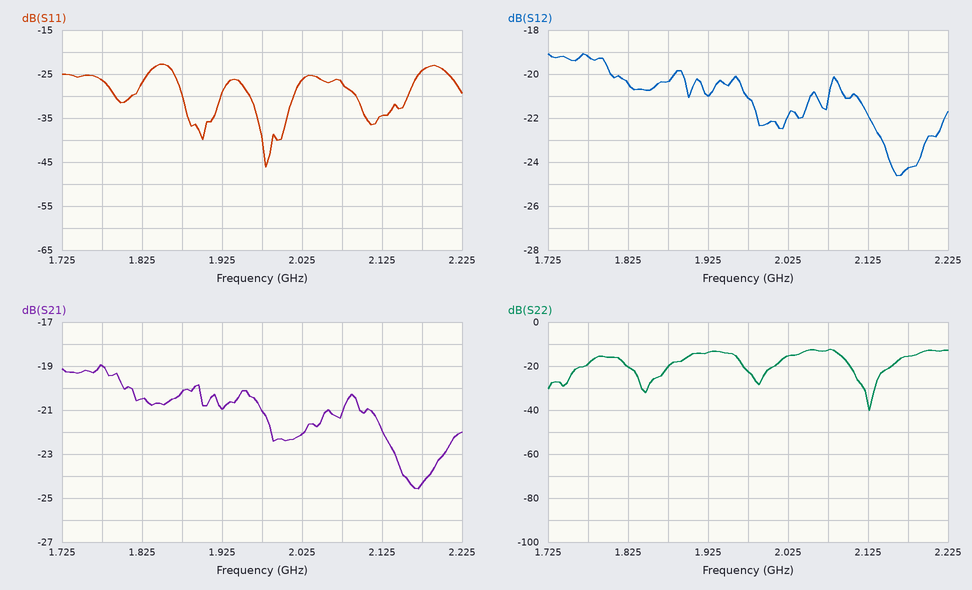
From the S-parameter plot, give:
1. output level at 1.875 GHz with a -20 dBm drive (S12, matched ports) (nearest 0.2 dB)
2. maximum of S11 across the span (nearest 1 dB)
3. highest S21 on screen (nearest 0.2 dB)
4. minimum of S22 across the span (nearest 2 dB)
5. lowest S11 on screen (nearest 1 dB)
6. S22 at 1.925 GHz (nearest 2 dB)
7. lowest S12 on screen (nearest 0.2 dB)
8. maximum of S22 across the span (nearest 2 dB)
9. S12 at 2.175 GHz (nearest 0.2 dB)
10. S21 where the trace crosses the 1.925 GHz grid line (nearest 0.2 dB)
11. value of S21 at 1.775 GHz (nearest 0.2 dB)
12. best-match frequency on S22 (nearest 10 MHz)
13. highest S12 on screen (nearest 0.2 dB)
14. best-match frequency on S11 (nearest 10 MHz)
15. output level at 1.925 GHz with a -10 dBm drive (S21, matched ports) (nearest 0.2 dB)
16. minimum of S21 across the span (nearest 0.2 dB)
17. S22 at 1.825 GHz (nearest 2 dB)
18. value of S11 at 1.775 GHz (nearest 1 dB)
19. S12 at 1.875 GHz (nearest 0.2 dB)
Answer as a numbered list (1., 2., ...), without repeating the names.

1. -40.4 dBm
2. -23 dB
3. -19.0 dB
4. -40 dB
5. -46 dB
6. -14 dB
7. -24.6 dB
8. -12 dB
9. -24.2 dB
10. -21.0 dB
11. -19.0 dB
12. 2.13 GHz
13. -19.0 dB
14. 1.98 GHz
15. -31.0 dBm
16. -24.6 dB
17. -20 dB
18. -26 dB
19. -20.4 dB
